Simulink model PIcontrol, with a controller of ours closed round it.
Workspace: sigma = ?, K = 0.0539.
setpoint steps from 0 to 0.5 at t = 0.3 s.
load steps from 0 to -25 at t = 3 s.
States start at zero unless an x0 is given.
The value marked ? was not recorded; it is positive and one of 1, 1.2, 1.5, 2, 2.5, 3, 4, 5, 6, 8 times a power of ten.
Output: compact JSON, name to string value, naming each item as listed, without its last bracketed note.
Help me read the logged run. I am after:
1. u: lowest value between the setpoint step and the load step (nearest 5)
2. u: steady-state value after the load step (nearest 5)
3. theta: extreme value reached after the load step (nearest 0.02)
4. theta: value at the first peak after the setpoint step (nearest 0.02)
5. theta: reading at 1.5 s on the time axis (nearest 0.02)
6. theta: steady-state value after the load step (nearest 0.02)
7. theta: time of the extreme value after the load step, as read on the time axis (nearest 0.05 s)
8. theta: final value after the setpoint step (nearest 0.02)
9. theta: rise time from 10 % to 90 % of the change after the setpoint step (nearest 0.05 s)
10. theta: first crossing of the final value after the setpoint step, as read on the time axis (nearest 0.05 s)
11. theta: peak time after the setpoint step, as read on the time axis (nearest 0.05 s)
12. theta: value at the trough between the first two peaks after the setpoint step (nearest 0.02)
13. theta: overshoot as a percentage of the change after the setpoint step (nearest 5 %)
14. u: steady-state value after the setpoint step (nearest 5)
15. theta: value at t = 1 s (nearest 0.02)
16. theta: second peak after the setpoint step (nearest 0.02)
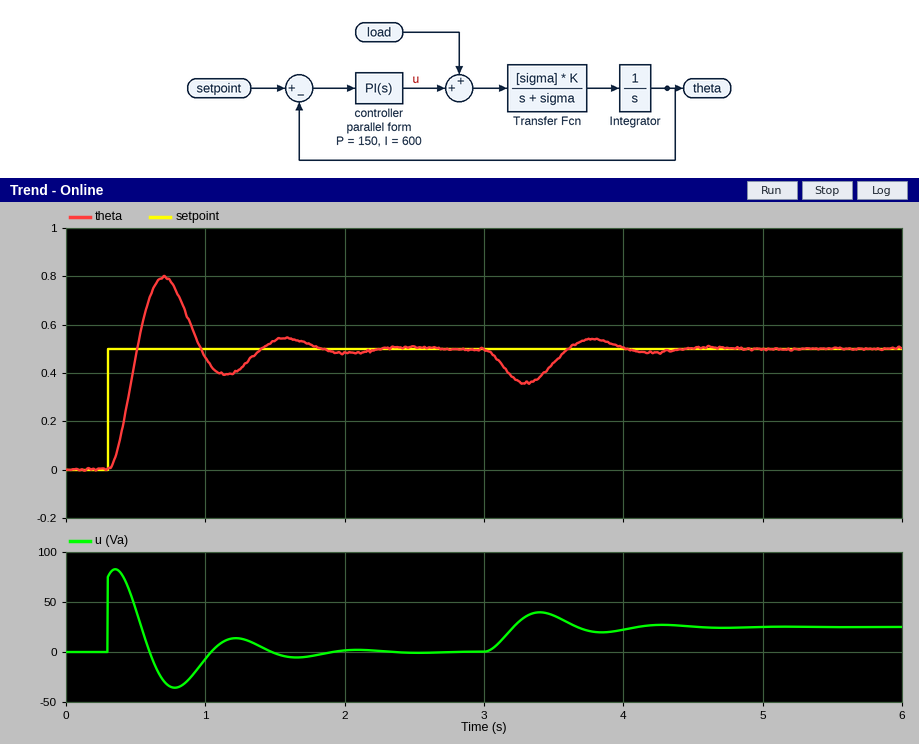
{"u: lowest value between the setpoint step and the load step": "-35", "u: steady-state value after the load step": "25", "theta: extreme value reached after the load step": "0.36", "theta: value at the first peak after the setpoint step": "0.80", "theta: reading at 1.5 s on the time axis": "0.54", "theta: steady-state value after the load step": "0.50", "theta: time of the extreme value after the load step, as read on the time axis": "3.30 s", "theta: final value after the setpoint step": "0.50", "theta: rise time from 10 % to 90 % of the change after the setpoint step": "0.15 s", "theta: first crossing of the final value after the setpoint step, as read on the time axis": "0.50 s", "theta: peak time after the setpoint step, as read on the time axis": "0.70 s", "theta: value at the trough between the first two peaks after the setpoint step": "0.40", "theta: overshoot as a percentage of the change after the setpoint step": "60 %", "u: steady-state value after the setpoint step": "0", "theta: value at t = 1 s": "0.46", "theta: second peak after the setpoint step": "0.54"}
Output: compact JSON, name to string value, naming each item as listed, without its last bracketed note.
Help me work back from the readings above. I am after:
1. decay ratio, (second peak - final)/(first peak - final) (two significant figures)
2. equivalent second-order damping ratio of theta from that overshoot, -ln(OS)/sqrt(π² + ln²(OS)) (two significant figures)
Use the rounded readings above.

{"decay ratio, (second peak - final)/(first peak - final)": "0.13", "equivalent second-order damping ratio of theta from that overshoot, -ln(OS)/sqrt(π² + ln²(OS))": "0.16"}
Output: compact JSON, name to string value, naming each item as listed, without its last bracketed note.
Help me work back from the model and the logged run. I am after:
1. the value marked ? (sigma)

{"the value marked ?": "10"}
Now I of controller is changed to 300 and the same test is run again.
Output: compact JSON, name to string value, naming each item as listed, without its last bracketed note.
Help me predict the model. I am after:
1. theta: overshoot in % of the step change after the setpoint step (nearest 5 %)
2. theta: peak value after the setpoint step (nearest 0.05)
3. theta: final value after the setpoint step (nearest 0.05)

{"theta: overshoot in % of the step change after the setpoint step": "40 %", "theta: peak value after the setpoint step": "0.70", "theta: final value after the setpoint step": "0.50"}
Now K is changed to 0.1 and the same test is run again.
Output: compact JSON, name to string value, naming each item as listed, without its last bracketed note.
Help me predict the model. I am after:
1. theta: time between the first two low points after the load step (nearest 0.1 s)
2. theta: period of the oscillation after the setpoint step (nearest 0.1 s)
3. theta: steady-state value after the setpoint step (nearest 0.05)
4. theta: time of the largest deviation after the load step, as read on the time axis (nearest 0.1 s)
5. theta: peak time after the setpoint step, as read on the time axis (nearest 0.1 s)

{"theta: time between the first two low points after the load step": "0.6 s", "theta: period of the oscillation after the setpoint step": "0.6 s", "theta: steady-state value after the setpoint step": "0.50", "theta: time of the largest deviation after the load step, as read on the time axis": "3.2 s", "theta: peak time after the setpoint step, as read on the time axis": "0.6 s"}
